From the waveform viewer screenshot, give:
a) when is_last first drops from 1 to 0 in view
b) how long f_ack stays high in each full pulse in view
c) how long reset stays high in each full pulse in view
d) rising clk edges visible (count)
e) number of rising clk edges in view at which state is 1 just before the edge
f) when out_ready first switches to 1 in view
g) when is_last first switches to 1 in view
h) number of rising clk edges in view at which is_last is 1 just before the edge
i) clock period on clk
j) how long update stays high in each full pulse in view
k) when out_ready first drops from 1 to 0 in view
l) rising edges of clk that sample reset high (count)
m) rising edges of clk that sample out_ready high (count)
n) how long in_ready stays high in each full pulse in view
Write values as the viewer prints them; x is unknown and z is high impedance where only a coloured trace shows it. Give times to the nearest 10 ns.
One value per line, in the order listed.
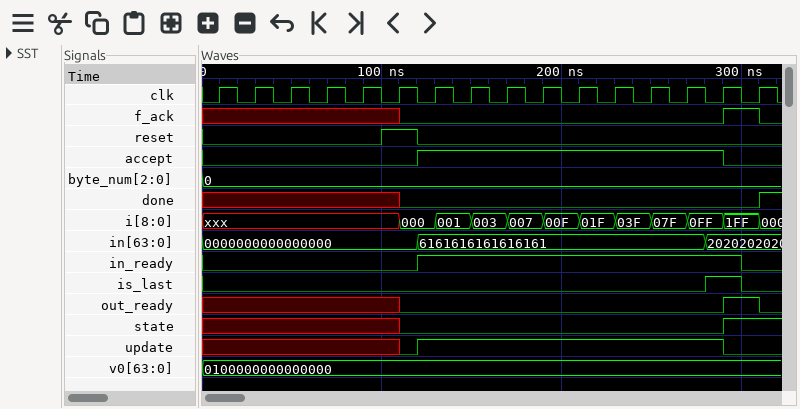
300 ns
20 ns
20 ns
16
1
290 ns
280 ns
1
20 ns
170 ns
310 ns
1
1
180 ns
